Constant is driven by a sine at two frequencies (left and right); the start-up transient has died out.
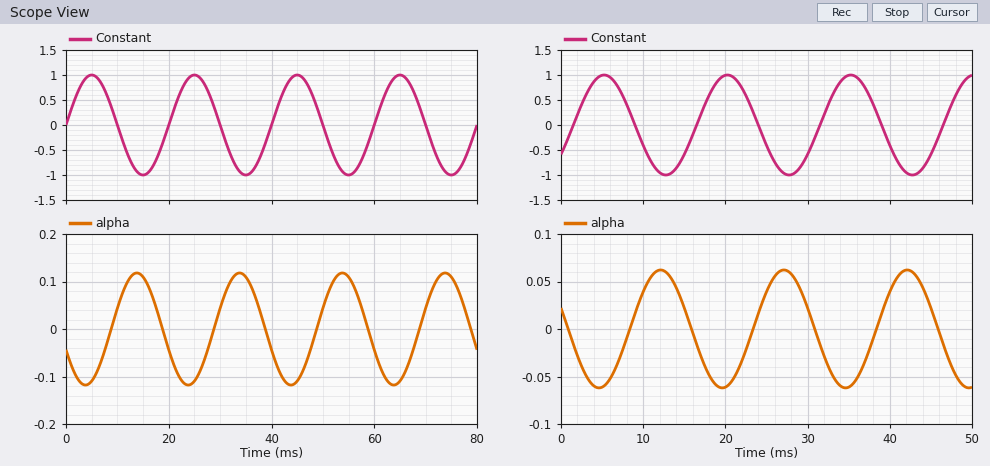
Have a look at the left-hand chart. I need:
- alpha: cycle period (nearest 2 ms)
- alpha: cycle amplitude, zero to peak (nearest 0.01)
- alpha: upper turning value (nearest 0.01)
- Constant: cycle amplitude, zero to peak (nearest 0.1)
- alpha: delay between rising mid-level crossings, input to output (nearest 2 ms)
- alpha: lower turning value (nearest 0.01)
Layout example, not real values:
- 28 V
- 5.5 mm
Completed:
- 20 ms
- 0.12
- 0.12
- 1.0
- 8 ms
- -0.12
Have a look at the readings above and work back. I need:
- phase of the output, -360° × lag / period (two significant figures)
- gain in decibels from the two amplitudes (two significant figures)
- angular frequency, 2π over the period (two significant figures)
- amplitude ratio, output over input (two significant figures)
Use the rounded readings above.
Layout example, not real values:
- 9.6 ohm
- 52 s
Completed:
- -140°
- -18 dB
- 0.31 rad/ms
- 0.12
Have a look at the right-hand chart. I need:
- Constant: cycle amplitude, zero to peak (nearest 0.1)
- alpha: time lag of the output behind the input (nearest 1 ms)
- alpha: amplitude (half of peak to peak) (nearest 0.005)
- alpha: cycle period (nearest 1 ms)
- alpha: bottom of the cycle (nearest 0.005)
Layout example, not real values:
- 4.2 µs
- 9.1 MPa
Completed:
- 1.0
- 7 ms
- 0.060
- 15 ms
- -0.060
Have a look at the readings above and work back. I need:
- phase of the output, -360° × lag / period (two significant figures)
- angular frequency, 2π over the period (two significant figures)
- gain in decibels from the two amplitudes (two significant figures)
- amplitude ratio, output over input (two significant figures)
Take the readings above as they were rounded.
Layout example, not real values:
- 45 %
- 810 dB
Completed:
- -170°
- 0.42 rad/ms
- -24 dB
- 0.060
